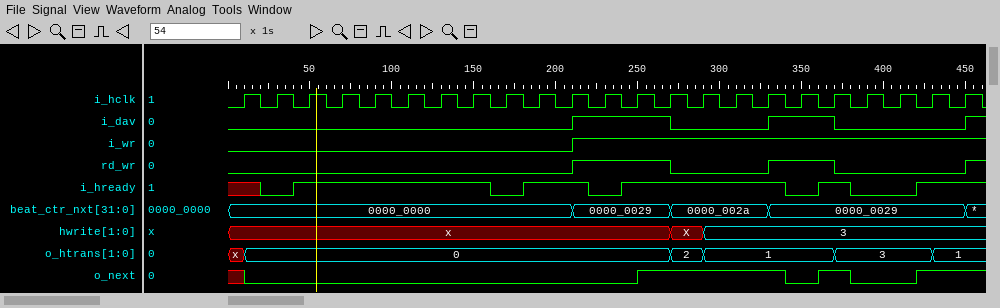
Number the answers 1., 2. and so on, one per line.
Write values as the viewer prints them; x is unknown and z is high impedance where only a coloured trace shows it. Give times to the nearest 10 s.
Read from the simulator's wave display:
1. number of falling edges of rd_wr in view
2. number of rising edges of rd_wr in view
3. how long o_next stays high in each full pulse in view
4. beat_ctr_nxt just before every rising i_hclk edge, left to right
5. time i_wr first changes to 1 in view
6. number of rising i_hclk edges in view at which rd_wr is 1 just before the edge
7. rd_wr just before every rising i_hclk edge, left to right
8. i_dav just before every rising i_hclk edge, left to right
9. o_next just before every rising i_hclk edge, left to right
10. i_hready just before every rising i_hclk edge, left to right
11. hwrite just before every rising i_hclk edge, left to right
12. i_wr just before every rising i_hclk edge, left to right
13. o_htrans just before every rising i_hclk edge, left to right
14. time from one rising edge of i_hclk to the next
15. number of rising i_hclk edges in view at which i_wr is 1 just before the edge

1. 2
2. 3
3. 90 s, 20 s
4. 0000_0000, 0000_0000, 0000_0000, 0000_0000, 0000_0000, 0000_0000, 0000_0000, 0000_0000, 0000_0000, 0000_0000, 0000_0000, 0000_0029, 0000_0029, 0000_0029, 0000_002a, 0000_002a, 0000_002a, 0000_0029, 0000_0029, 0000_0029, 0000_0029, 0000_0029, 0000_0029
5. 210 s
6. 5
7. 0 0 0 0 0 0 0 0 0 0 0 1 1 1 0 0 0 1 1 0 0 0 0
8. 0 0 0 0 0 0 0 0 0 0 0 1 1 1 0 0 0 1 1 0 0 0 0
9. x 0 0 0 0 0 0 0 0 0 0 0 0 1 1 1 1 0 1 0 0 1 1
10. x 0 1 1 1 1 1 1 0 1 1 0 1 1 1 1 1 0 1 0 0 1 1
11. x, x, x, x, x, x, x, x, x, x, x, x, x, x, X, 3, 3, 3, 3, 3, 3, 3, 3
12. 0 0 0 0 0 0 0 0 0 0 0 1 1 1 1 1 1 1 1 1 1 1 1
13. x, 0, 0, 0, 0, 0, 0, 0, 0, 0, 0, 0, 0, 0, 2, 1, 1, 1, 1, 3, 3, 3, 1
14. 20 s
15. 12
